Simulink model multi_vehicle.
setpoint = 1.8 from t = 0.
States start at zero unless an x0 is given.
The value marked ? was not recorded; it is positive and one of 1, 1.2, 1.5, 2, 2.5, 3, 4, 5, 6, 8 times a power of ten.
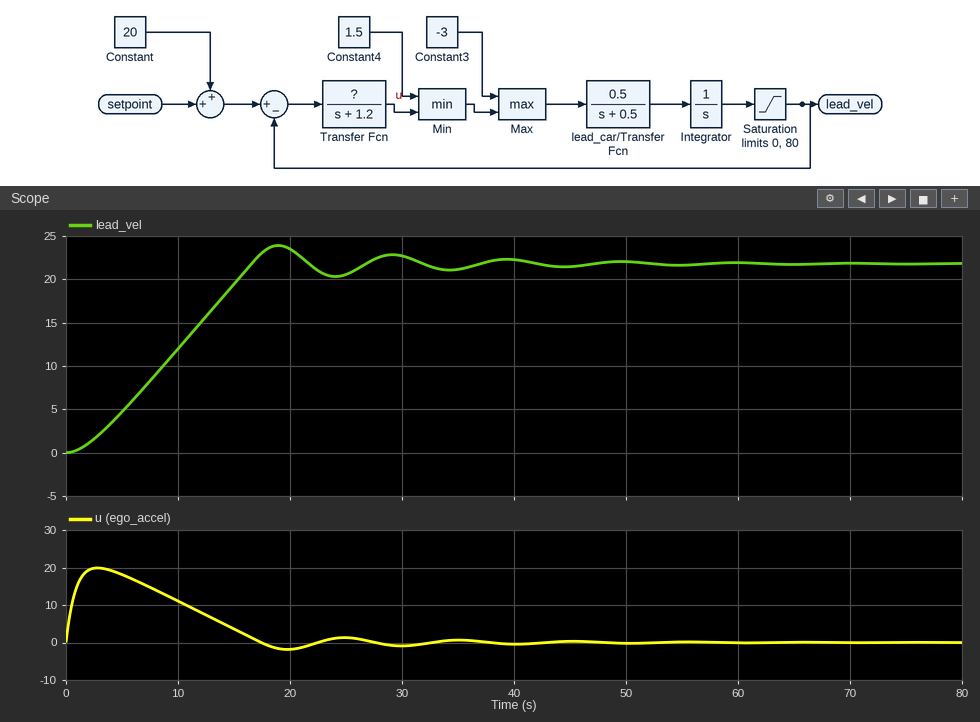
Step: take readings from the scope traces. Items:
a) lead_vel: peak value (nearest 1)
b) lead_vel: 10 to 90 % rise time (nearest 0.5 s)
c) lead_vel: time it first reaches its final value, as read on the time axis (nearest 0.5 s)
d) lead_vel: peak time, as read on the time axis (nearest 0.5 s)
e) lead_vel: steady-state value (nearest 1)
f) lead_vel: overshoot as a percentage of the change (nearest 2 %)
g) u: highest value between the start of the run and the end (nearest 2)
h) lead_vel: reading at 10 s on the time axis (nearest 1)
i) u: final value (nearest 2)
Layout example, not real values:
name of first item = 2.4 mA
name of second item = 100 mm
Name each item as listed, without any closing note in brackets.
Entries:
lead_vel: peak value = 24
lead_vel: 10 to 90 % rise time = 12.0 s
lead_vel: time it first reaches its final value, as read on the time axis = 16.5 s
lead_vel: peak time, as read on the time axis = 19.0 s
lead_vel: steady-state value = 22
lead_vel: overshoot as a percentage of the change = 10 %
u: highest value between the start of the run and the end = 20
lead_vel: reading at 10 s on the time axis = 12
u: final value = 0
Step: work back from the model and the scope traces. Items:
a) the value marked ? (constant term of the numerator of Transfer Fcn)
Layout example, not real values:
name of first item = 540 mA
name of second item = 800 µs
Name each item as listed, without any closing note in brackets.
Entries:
the value marked ? = 1.2
